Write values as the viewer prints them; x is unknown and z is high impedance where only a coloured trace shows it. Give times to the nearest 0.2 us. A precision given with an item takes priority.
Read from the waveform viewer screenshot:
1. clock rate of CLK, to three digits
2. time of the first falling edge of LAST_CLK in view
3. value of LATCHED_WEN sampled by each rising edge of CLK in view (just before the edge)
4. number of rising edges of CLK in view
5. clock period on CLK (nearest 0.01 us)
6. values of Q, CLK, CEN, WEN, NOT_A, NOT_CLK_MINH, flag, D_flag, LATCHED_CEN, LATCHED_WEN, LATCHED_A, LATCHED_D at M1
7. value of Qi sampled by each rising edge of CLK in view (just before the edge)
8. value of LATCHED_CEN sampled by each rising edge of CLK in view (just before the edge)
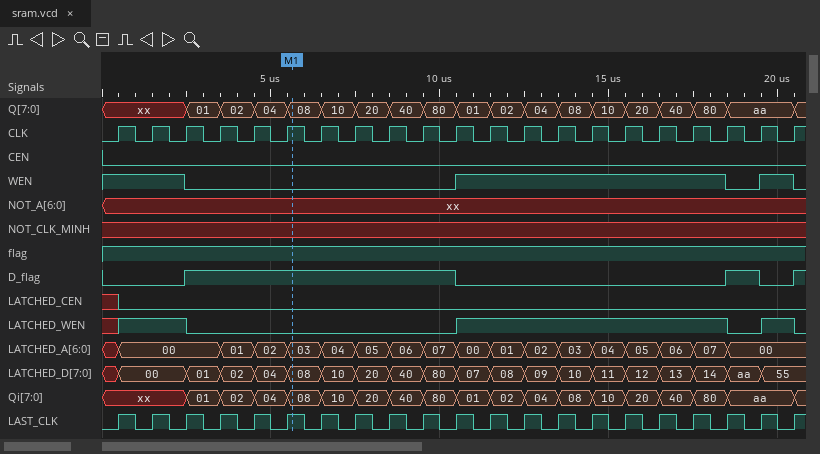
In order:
1.00 MHz
1 us
x 1 1 0 0 0 0 0 0 0 0 1 1 1 1 1 1 1 1 0 1
21
1 us
Q=08, CLK=1, CEN=0, WEN=0, NOT_A=xx, NOT_CLK_MINH=x, flag=1, D_flag=1, LATCHED_CEN=0, LATCHED_WEN=0, LATCHED_A=03, LATCHED_D=08
xx, xx, xx, 01, 02, 04, 08, 10, 20, 40, 80, 01, 02, 04, 08, 10, 20, 40, 80, aa, aa
x 0 0 0 0 0 0 0 0 0 0 0 0 0 0 0 0 0 0 0 0
